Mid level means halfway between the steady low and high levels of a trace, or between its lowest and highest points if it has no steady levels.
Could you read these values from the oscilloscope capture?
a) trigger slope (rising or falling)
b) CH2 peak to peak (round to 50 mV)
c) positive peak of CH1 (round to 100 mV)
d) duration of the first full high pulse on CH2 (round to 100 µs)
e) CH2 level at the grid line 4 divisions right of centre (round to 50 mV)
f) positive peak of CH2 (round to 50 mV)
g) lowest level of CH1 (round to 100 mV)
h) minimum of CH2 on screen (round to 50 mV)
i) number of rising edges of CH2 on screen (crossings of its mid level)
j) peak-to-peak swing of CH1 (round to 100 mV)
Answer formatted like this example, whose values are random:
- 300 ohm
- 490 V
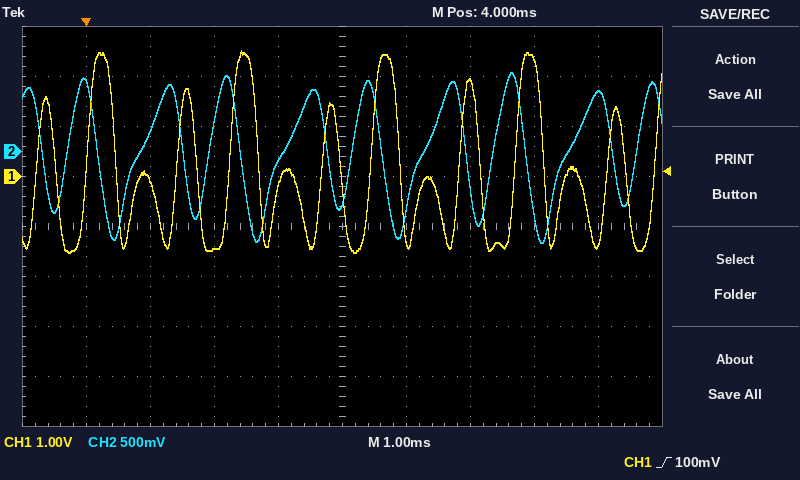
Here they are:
- rising
- 1.70 V
- 2.5 V
- 500 µs
- 600 mV
- 800 mV
- -1.5 V
- -900 mV
- 9
- 4.0 V
